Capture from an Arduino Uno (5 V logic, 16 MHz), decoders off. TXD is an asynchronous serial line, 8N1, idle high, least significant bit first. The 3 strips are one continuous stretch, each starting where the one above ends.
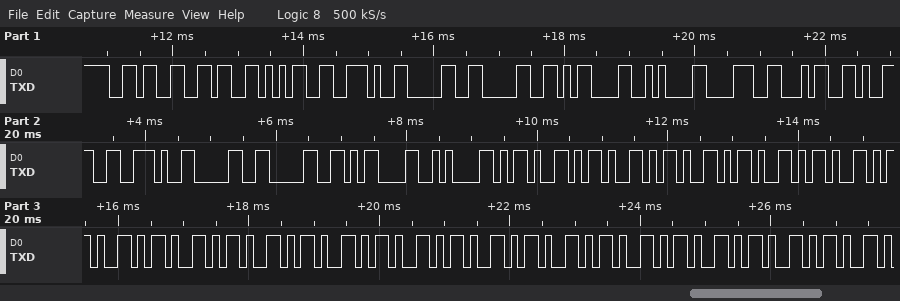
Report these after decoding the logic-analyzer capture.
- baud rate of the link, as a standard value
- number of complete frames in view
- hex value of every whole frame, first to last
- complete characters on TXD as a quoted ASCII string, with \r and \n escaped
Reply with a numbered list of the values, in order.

1. 9600 baud
2. 32
3. 36 36 35 2E 30 30 0D 0A 38 34 39 2E 30 30 0D 0A 2D 2D 2D 2D 2D 2D 2D 2D 2D 2D 2D 2D 2D 2D 2D 2D
4. "665.00\r\n849.00\r\n----------------"
